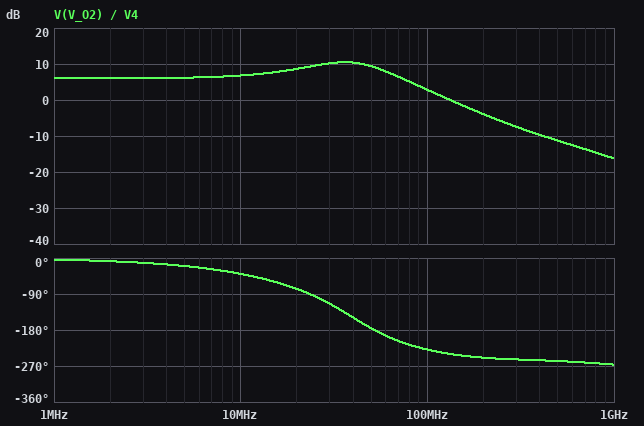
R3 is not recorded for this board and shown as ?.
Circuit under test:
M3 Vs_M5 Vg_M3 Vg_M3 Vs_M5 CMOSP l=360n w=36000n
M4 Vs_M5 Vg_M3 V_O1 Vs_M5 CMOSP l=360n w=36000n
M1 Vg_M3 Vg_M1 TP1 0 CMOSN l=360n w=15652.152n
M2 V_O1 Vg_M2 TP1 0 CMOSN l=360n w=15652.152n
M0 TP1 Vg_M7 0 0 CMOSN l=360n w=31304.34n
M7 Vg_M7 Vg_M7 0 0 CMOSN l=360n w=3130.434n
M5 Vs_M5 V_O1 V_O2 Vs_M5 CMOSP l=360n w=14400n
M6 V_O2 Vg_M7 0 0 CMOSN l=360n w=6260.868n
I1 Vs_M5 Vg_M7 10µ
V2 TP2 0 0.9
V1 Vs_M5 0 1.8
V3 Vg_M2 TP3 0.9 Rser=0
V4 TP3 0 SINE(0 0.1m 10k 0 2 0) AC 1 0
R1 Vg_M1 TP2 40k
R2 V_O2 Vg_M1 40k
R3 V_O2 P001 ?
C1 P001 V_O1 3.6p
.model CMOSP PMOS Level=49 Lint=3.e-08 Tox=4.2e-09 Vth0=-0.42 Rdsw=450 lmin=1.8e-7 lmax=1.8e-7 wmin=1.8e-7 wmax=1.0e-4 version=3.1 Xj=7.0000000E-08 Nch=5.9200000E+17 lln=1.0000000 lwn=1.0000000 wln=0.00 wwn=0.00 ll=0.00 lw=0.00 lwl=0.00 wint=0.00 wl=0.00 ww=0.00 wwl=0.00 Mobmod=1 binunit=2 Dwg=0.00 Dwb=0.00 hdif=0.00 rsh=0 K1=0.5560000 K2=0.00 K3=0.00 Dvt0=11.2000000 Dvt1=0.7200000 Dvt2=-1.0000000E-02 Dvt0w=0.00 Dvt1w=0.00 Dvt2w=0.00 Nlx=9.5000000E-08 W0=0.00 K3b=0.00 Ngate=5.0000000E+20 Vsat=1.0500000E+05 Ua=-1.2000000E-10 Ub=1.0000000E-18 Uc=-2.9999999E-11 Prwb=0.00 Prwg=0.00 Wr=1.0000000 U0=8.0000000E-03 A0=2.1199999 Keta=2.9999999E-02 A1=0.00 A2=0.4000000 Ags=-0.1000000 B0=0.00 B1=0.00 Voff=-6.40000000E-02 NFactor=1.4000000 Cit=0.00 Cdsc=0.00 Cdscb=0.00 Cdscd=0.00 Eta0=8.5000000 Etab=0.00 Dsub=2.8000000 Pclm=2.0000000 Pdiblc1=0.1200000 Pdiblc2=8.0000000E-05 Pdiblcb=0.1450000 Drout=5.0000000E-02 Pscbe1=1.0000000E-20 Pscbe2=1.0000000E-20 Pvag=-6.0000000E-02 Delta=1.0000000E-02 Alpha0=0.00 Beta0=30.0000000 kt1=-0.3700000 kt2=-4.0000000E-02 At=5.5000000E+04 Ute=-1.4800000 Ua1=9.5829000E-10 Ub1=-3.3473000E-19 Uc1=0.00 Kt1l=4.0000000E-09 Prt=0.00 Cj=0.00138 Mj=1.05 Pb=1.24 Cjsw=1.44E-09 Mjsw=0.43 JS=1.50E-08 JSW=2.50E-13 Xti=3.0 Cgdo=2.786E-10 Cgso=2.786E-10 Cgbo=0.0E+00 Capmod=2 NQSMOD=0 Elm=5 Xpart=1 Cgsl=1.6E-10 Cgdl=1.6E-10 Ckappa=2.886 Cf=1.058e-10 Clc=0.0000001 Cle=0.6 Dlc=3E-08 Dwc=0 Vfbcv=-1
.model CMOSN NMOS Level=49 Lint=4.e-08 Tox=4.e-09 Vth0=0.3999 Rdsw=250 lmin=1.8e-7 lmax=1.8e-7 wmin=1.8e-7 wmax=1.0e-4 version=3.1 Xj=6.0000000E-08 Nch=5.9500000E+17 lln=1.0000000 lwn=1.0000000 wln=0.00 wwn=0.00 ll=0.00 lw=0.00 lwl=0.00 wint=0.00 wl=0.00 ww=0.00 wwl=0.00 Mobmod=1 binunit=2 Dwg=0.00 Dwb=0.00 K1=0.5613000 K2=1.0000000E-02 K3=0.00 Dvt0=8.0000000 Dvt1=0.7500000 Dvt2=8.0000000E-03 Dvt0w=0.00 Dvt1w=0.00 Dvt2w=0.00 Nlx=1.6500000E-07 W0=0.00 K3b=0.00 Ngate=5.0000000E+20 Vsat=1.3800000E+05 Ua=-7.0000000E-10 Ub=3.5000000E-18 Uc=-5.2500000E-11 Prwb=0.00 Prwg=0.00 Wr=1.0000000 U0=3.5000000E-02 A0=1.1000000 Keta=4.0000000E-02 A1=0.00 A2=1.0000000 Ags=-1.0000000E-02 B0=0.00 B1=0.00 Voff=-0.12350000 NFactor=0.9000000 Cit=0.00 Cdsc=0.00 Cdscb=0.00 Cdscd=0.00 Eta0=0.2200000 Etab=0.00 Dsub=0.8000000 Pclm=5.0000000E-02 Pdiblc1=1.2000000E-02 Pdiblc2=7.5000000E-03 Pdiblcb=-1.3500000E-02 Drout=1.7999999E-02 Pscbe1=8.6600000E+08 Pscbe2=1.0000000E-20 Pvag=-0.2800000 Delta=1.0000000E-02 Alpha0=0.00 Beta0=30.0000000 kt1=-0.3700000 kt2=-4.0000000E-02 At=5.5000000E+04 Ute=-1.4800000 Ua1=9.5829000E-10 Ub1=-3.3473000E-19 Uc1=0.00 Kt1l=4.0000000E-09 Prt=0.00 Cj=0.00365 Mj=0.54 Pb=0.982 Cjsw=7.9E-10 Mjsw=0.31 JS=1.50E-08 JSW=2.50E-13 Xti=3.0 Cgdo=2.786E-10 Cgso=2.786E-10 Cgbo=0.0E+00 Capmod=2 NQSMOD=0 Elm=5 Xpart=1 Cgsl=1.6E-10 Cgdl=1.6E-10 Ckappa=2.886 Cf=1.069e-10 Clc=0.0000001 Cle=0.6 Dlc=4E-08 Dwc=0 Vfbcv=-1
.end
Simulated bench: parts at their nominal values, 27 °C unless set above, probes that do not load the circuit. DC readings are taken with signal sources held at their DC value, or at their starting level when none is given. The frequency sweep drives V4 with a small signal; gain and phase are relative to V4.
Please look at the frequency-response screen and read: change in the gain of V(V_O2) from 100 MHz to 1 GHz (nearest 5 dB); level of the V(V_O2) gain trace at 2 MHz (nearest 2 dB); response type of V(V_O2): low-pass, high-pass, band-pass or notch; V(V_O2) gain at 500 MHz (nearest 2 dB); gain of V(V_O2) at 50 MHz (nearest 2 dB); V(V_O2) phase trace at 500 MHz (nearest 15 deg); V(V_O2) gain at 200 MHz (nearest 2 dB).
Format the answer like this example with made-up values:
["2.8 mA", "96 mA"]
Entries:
["-20 dB", "6 dB", "low-pass", "-12 dB", "10 dB", "-255 deg", "-4 dB"]
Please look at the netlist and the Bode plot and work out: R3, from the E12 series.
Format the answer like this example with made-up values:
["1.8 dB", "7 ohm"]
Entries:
["1.2 kΩ"]
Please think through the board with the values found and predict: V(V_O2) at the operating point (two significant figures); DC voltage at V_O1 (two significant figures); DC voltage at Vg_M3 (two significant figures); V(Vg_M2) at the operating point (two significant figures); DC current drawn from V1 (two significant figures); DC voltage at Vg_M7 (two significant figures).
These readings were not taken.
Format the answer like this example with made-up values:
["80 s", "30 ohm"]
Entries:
["900 mV", "1.2 V", "1.2 V", "900 mV", "120 µA", "570 mV"]
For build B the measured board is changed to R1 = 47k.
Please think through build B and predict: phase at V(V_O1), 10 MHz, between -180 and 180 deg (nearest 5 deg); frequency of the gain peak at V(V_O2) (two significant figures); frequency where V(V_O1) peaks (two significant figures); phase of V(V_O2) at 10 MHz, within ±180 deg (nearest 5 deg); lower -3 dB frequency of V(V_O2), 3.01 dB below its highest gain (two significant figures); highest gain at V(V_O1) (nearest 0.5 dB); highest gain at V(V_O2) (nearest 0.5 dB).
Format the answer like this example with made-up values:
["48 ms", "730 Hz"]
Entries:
["-110 deg", "38 MHz", "41 MHz", "-35 deg", "20 MHz", "15.0 dB", "11.5 dB"]
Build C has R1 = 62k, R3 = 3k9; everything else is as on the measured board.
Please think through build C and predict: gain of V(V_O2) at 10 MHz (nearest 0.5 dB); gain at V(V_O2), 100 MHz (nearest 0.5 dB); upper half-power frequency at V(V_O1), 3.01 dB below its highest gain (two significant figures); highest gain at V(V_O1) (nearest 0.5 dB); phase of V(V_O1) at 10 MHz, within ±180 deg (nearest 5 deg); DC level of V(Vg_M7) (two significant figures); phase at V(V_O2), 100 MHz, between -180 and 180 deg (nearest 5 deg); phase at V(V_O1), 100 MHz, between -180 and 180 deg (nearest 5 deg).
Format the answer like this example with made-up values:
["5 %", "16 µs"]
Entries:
["2.5 dB", "-6.0 dB", "260 MHz", "4.5 dB", "-135 deg", "570 mV", "-55 deg", "165 deg"]
